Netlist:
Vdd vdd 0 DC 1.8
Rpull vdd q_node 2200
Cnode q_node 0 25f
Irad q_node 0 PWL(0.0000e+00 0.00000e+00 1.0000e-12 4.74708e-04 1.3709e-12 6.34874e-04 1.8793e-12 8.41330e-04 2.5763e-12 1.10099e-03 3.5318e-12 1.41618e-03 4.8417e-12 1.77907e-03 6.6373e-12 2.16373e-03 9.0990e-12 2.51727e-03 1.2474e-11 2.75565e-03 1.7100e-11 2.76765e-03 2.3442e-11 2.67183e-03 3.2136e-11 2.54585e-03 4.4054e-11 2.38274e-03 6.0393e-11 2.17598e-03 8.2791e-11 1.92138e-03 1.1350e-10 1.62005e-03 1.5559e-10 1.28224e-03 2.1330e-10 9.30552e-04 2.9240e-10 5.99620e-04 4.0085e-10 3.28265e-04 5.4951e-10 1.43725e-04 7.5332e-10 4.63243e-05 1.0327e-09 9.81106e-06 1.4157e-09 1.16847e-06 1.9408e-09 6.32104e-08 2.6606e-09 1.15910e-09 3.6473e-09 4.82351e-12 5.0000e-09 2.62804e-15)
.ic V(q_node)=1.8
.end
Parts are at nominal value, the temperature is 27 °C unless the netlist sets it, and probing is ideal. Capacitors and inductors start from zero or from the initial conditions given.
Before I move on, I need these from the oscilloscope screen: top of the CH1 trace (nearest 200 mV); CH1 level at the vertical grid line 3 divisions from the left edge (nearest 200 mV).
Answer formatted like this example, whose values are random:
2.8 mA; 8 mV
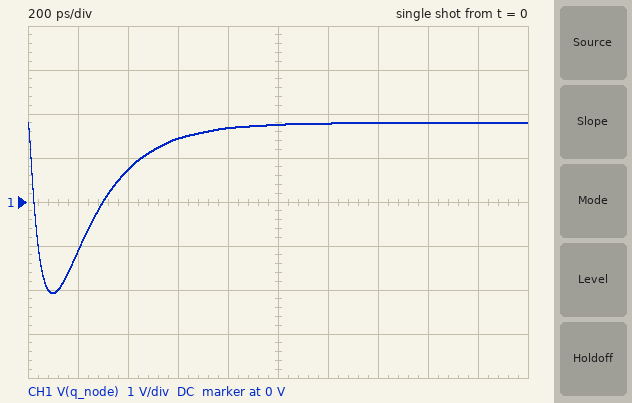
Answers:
1.8 V; 1.4 V
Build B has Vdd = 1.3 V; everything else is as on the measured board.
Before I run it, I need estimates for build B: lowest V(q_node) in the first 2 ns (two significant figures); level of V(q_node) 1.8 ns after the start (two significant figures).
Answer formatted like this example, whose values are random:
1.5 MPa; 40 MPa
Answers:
-2.5 V; 1.3 V
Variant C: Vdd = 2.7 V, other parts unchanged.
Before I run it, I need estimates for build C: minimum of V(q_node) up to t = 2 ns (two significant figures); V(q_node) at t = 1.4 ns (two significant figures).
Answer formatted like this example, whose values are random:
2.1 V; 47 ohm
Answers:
-1.3 V; 2.7 V
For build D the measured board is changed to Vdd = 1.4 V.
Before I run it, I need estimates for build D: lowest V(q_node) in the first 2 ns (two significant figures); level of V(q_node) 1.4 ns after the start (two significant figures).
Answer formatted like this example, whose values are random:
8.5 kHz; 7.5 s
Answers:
-2.4 V; 1.4 V
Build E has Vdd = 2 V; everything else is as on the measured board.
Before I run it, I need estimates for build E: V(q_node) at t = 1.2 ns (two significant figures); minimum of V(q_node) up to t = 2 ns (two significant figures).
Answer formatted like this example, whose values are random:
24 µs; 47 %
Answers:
2.0 V; -1.9 V
